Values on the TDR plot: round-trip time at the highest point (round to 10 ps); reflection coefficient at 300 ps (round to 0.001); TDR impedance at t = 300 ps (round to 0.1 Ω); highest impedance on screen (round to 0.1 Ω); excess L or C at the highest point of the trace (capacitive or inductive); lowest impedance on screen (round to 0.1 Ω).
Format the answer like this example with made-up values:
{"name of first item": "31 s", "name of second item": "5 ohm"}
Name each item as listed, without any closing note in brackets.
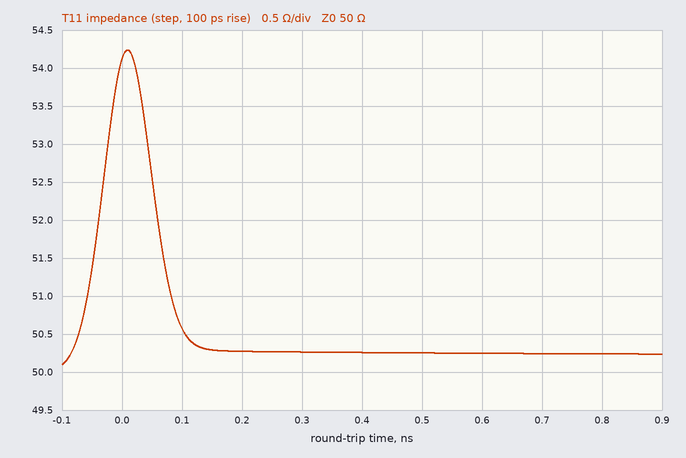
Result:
{"round-trip time at the highest point": "10 ps", "reflection coefficient at 300 ps": "+0.003", "TDR impedance at t = 300 ps": "50.3 Ω", "highest impedance on screen": "54.2 Ω", "excess L or C at the highest point of the trace": "inductive", "lowest impedance on screen": "50.1 Ω"}
